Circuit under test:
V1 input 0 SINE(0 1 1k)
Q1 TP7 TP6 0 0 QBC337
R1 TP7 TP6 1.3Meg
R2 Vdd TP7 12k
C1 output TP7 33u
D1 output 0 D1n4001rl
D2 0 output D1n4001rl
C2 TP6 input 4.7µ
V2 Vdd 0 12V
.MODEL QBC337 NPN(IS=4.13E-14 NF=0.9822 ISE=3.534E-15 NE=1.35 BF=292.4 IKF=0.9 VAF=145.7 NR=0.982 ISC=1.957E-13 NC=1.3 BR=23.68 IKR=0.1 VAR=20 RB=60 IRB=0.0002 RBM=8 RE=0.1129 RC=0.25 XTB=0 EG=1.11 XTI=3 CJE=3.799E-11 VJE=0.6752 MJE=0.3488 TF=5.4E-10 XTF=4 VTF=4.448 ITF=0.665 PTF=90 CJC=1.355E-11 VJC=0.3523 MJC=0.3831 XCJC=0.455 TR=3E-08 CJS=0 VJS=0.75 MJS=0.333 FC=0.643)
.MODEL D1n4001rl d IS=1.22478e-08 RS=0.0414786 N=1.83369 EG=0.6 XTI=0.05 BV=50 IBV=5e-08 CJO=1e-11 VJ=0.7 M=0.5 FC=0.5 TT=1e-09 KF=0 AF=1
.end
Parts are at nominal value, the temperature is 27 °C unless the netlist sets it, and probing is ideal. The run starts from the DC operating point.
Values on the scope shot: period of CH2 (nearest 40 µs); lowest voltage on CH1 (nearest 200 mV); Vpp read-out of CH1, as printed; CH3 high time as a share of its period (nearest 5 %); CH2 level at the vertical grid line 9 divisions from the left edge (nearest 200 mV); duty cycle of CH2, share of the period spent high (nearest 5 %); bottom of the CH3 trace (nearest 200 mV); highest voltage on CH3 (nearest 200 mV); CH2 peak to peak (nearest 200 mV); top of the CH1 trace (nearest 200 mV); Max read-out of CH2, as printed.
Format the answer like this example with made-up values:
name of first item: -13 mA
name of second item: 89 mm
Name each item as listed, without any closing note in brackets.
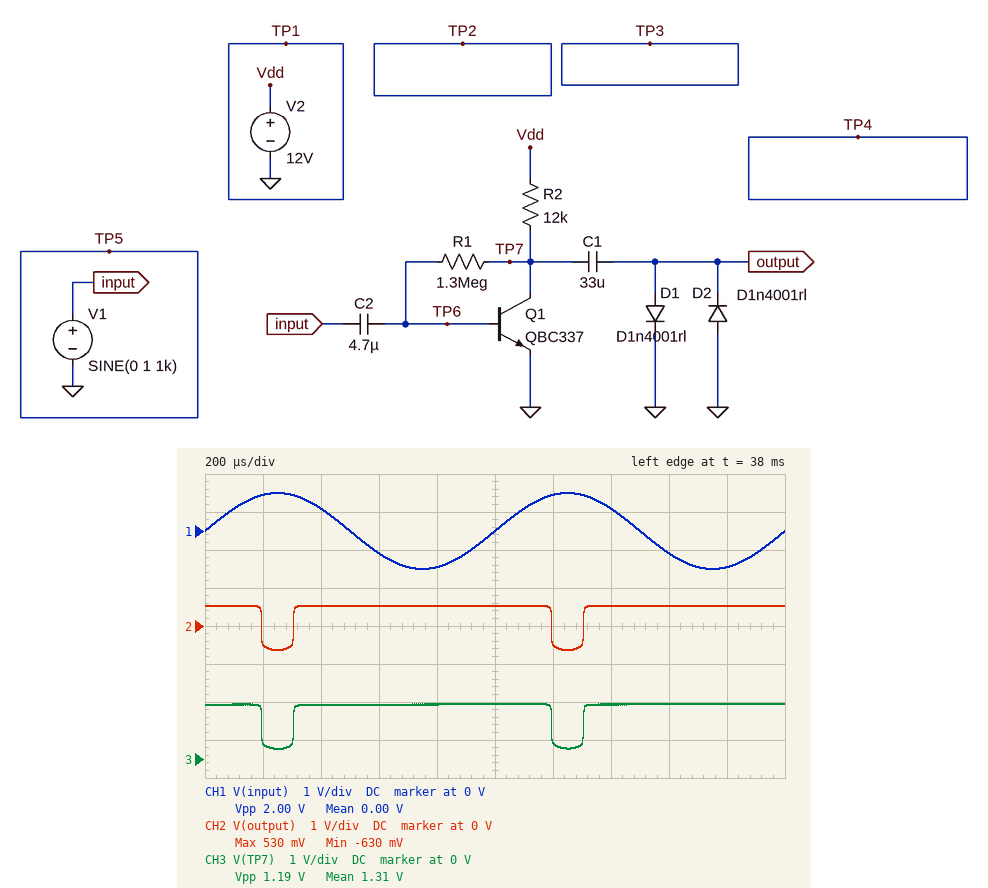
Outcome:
period of CH2: 1.00 ms
lowest voltage on CH1: -1.0 V
Vpp read-out of CH1, as printed: 2.00 V
CH3 high time as a share of its period: 90 %
CH2 level at the vertical grid line 9 divisions from the left edge: 600 mV
duty cycle of CH2, share of the period spent high: 90 %
bottom of the CH3 trace: 200 mV
highest voltage on CH3: 1.4 V
CH2 peak to peak: 1.2 V
top of the CH1 trace: 1.0 V
Max read-out of CH2, as printed: 530 mV
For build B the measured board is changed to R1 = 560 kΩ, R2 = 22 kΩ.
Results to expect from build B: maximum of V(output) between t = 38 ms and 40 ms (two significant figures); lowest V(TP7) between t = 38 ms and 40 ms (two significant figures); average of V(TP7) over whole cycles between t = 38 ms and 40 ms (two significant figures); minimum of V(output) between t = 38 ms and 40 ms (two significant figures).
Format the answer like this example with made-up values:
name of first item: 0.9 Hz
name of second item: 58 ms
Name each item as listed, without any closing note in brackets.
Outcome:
maximum of V(output) between t = 38 ms and 40 ms: 500 mV
lowest V(TP7) between t = 38 ms and 40 ms: 85 mV
average of V(TP7) over whole cycles between t = 38 ms and 40 ms: 1.1 V
minimum of V(output) between t = 38 ms and 40 ms: -620 mV
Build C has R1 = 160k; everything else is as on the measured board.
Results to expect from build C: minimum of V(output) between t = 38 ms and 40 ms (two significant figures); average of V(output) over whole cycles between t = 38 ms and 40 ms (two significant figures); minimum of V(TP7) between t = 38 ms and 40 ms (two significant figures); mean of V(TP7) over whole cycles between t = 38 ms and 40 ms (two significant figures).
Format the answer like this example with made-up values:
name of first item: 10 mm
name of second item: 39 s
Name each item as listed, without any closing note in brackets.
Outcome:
minimum of V(output) between t = 38 ms and 40 ms: -650 mV
average of V(output) over whole cycles between t = 38 ms and 40 ms: 390 mV
minimum of V(TP7) between t = 38 ms and 40 ms: 54 mV
mean of V(TP7) over whole cycles between t = 38 ms and 40 ms: 1.1 V
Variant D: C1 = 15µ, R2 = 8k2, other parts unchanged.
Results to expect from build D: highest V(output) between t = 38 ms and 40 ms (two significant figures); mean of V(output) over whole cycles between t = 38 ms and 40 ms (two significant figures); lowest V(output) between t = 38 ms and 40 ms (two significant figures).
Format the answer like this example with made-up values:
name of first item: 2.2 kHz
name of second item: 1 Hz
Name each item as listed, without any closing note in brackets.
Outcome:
highest V(output) between t = 38 ms and 40 ms: 550 mV
mean of V(output) over whole cycles between t = 38 ms and 40 ms: 420 mV
lowest V(output) between t = 38 ms and 40 ms: -650 mV
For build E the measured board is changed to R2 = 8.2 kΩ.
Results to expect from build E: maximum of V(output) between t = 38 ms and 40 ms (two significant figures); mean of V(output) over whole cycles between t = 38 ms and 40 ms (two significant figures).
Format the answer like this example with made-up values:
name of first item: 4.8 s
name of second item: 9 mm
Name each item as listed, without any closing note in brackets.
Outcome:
maximum of V(output) between t = 38 ms and 40 ms: 550 mV
mean of V(output) over whole cycles between t = 38 ms and 40 ms: 420 mV
